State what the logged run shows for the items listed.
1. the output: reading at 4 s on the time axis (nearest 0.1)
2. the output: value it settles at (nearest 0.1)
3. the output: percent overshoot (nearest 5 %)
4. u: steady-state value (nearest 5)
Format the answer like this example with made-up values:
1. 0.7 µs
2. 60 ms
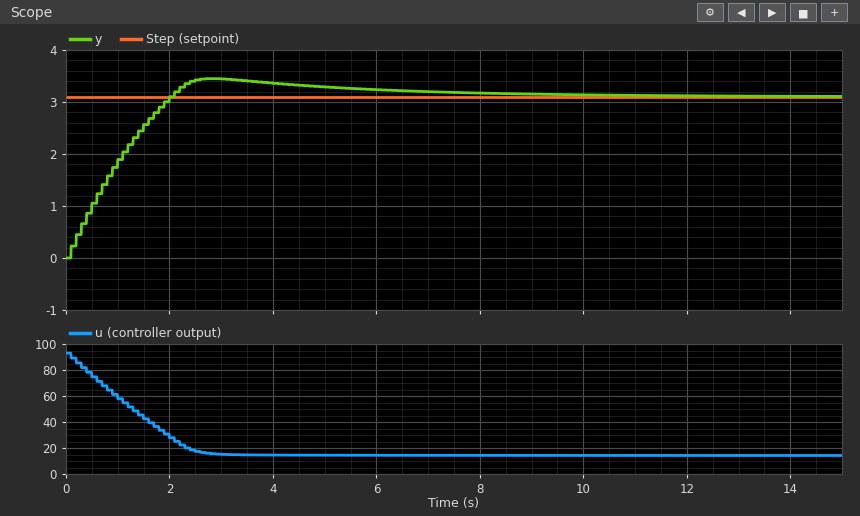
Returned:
1. 3.4
2. 3.1
3. 10 %
4. 15
